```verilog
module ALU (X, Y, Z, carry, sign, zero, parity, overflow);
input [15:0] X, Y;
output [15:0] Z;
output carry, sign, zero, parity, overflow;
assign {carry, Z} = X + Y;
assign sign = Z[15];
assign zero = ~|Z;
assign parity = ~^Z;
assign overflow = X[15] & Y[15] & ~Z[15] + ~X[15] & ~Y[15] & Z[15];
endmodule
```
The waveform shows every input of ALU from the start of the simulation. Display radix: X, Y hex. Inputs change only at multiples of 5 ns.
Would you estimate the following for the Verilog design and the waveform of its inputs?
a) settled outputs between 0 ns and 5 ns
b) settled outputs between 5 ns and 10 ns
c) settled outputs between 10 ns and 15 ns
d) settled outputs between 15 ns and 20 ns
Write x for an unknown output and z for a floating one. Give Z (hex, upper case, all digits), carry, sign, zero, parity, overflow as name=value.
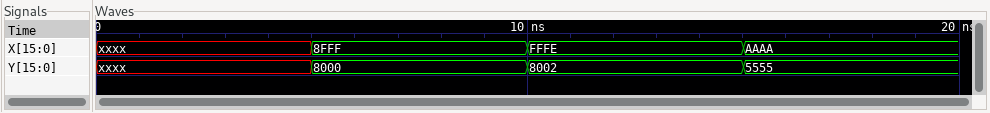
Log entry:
Z=x, carry=x, sign=x, zero=x, parity=x, overflow=x
Z=0FFF, carry=1, sign=0, zero=0, parity=1, overflow=0
Z=8000, carry=1, sign=1, zero=0, parity=0, overflow=0
Z=FFFF, carry=0, sign=1, zero=0, parity=1, overflow=0
